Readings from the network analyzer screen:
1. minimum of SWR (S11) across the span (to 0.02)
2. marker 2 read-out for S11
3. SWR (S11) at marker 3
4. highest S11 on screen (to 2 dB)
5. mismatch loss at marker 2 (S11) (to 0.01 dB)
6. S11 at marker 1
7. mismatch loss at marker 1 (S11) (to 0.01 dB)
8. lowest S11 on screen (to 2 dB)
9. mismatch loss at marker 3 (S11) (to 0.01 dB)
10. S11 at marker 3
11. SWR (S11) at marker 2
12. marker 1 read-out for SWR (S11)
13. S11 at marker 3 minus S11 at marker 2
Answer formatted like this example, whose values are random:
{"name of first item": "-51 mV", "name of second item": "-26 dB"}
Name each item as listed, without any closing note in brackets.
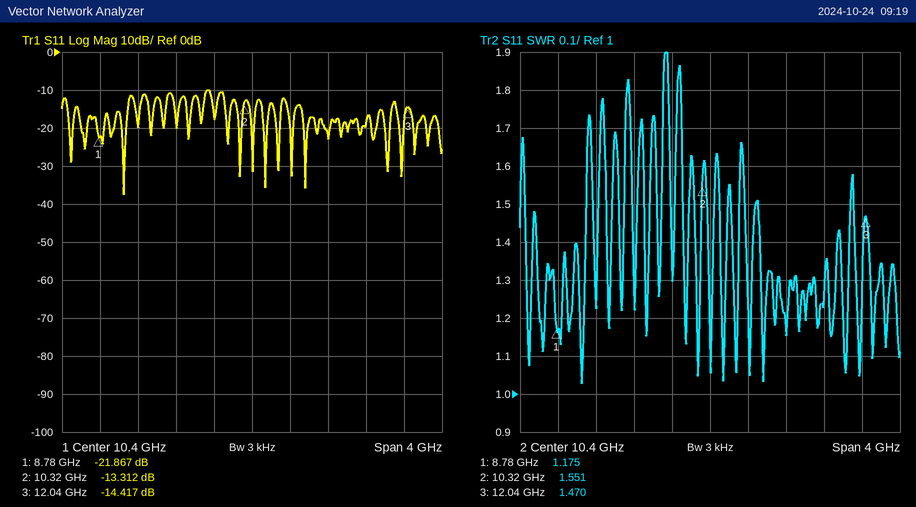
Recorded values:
{"minimum of SWR (S11) across the span": "1.02", "marker 2 read-out for S11": "-13.312 dB", "SWR (S11) at marker 3": "1.470", "highest S11 on screen": "-10 dB", "mismatch loss at marker 2 (S11)": "0.21 dB", "S11 at marker 1": "-21.867 dB", "mismatch loss at marker 1 (S11)": "0.03 dB", "lowest S11 on screen": "-38 dB", "mismatch loss at marker 3 (S11)": "0.16 dB", "S11 at marker 3": "-14.417 dB", "SWR (S11) at marker 2": "1.551", "marker 1 read-out for SWR": "1.175", "S11 at marker 3 minus S11 at marker 2": "-1.105 dB"}
